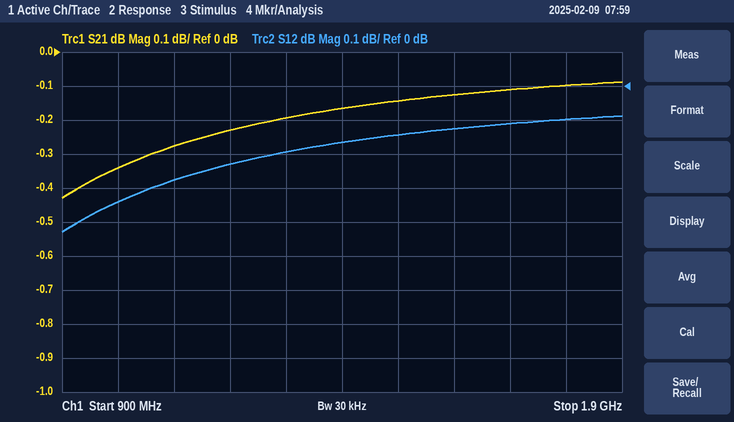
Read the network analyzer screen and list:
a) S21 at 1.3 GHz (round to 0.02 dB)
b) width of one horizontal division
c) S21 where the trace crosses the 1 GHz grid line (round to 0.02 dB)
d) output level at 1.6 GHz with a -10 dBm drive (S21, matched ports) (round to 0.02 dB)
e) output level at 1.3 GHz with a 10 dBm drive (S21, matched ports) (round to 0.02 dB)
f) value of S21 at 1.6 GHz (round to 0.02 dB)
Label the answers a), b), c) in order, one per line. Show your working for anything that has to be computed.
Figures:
a) -0.20 dB
b) 100 MHz
c) -0.34 dB
d) -10 dBm + (-0.12 dB) = -10.12 dBm
e) 10 dBm + (-0.20 dB) = 9.80 dBm
f) -0.12 dB
